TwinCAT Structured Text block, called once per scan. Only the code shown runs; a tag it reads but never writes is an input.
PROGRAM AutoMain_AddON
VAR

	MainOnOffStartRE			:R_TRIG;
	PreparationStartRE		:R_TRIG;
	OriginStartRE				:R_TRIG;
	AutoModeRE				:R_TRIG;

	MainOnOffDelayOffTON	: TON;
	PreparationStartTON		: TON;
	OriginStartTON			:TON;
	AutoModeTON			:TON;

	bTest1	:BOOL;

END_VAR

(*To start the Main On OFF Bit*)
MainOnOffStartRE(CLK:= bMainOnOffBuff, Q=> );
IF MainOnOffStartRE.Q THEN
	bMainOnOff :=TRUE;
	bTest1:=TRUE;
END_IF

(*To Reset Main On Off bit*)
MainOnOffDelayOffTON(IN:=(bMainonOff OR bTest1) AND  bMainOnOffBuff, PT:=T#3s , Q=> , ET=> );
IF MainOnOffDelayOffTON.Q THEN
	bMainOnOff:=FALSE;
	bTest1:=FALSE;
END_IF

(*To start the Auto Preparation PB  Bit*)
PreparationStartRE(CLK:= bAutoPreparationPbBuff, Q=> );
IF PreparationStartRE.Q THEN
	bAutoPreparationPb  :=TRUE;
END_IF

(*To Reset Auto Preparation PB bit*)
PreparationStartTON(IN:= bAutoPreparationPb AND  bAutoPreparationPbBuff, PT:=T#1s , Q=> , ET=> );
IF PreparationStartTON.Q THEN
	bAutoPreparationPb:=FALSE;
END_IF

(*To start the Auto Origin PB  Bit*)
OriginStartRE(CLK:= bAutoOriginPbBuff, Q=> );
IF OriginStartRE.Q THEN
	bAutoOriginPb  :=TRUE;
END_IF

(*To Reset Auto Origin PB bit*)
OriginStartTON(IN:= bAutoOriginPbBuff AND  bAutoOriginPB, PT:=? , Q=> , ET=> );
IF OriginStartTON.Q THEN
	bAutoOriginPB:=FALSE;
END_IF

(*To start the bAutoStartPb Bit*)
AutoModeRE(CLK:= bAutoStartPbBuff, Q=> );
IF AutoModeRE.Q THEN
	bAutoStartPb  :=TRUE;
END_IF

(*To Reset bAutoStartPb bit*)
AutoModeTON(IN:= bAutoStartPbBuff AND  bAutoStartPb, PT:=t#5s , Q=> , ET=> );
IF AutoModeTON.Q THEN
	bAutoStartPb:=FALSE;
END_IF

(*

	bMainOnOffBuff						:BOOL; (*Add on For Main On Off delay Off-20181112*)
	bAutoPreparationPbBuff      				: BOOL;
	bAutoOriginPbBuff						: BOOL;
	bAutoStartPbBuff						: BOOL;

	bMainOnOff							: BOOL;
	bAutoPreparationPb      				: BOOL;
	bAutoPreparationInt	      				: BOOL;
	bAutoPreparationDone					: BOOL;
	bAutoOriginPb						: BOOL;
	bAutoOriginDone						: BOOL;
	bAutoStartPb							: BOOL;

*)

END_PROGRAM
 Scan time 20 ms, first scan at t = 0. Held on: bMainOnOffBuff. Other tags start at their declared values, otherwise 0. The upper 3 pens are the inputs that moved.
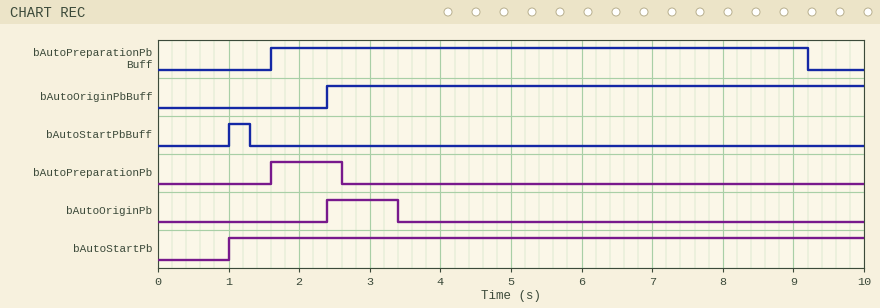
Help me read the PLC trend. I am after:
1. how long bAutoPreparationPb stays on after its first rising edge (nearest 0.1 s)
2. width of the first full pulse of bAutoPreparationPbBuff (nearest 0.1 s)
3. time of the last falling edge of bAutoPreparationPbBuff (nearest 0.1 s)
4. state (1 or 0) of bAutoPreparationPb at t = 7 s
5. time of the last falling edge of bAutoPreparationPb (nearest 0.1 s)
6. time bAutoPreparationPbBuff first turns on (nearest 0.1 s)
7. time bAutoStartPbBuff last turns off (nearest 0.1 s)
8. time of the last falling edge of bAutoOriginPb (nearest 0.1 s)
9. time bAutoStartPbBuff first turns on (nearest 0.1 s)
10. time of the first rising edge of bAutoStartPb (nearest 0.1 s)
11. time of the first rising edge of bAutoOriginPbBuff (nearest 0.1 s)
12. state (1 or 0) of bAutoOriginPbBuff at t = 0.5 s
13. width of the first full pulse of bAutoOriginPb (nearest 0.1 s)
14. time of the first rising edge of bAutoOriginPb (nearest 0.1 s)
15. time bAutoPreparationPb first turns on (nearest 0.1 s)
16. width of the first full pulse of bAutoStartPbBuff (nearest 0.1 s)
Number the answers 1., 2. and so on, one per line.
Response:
1. 1.0 s
2. 7.6 s
3. 9.2 s
4. 0
5. 2.6 s
6. 1.6 s
7. 1.3 s
8. 3.4 s
9. 1.0 s
10. 1.0 s
11. 2.4 s
12. 0
13. 1.0 s
14. 2.4 s
15. 1.6 s
16. 0.3 s
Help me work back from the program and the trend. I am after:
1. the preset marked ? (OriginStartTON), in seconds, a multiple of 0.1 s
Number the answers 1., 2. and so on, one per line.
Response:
1. 1.0 s
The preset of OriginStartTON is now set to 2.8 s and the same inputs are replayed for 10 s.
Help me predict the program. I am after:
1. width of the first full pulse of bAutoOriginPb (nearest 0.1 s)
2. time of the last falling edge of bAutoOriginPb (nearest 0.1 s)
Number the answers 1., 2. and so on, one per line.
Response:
1. 2.8 s
2. 5.2 s
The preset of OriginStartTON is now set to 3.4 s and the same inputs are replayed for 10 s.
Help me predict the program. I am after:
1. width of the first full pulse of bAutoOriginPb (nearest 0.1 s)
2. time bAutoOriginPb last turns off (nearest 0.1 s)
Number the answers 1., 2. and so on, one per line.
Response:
1. 3.4 s
2. 5.8 s
